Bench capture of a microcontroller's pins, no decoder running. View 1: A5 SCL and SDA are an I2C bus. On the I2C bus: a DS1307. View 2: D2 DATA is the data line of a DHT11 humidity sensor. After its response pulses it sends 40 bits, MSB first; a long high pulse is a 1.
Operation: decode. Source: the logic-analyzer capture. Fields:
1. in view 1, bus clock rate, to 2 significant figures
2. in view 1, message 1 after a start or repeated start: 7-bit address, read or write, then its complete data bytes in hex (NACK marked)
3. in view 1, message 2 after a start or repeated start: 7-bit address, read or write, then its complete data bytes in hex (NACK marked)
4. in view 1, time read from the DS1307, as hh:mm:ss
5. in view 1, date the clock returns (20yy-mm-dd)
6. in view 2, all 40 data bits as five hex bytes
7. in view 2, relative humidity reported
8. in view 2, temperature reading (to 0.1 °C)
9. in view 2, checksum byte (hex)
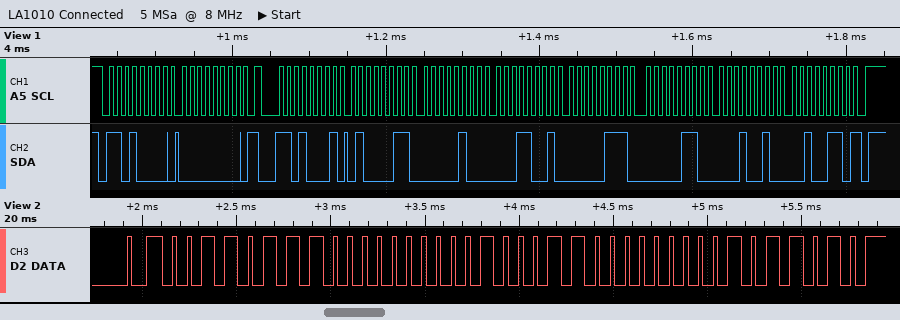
100 kHz
0x68 write: 00
0x68 read: 43 04 19 07 06 12 26 NACK
19:04:43
2026-12-06
37 00 23 00 5A
55 %
35.0 °C
0x5A
